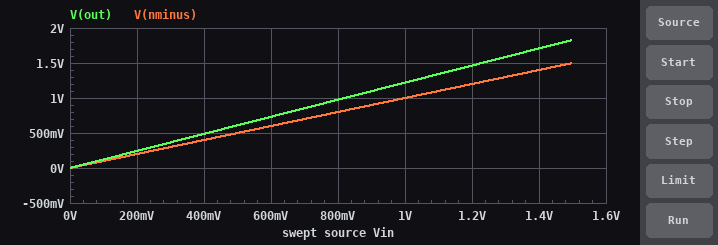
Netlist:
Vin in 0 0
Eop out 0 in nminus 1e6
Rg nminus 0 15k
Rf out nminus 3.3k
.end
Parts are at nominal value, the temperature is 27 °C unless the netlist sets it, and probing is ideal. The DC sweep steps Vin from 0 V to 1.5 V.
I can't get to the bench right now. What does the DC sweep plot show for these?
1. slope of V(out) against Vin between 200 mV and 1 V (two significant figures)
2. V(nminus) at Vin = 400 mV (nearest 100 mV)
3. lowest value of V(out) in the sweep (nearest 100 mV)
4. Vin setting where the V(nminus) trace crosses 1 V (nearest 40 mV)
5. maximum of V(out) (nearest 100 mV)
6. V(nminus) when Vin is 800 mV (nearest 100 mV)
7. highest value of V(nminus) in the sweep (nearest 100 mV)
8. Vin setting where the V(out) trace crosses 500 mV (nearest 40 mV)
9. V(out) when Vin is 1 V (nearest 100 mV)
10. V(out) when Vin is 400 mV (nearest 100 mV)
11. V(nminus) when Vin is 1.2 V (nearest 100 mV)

1.2 V/V
400 mV
0 V
1.00 V
1.8 V
800 mV
1.5 V
400 mV
1.2 V
500 mV
1.2 V
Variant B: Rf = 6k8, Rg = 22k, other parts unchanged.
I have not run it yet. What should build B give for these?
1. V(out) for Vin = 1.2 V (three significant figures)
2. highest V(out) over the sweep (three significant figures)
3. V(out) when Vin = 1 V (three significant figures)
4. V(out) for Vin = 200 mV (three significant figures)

1.57 V
1.96 V
1.31 V
262 mV
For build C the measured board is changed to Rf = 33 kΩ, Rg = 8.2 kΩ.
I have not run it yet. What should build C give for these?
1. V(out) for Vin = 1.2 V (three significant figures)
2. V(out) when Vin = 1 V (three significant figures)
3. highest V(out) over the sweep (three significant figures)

6.03 V
5.02 V
7.54 V
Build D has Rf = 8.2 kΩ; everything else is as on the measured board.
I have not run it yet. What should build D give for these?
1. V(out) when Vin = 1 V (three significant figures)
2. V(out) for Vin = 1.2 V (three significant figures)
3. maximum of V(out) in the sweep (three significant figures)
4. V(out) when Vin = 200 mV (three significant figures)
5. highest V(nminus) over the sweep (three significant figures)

1.55 V
1.86 V
2.32 V
309 mV
1.50 V
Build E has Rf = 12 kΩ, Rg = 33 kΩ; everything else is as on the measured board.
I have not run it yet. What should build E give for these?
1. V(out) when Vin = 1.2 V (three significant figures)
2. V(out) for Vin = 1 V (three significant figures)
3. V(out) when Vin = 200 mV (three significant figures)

1.64 V
1.36 V
273 mV
